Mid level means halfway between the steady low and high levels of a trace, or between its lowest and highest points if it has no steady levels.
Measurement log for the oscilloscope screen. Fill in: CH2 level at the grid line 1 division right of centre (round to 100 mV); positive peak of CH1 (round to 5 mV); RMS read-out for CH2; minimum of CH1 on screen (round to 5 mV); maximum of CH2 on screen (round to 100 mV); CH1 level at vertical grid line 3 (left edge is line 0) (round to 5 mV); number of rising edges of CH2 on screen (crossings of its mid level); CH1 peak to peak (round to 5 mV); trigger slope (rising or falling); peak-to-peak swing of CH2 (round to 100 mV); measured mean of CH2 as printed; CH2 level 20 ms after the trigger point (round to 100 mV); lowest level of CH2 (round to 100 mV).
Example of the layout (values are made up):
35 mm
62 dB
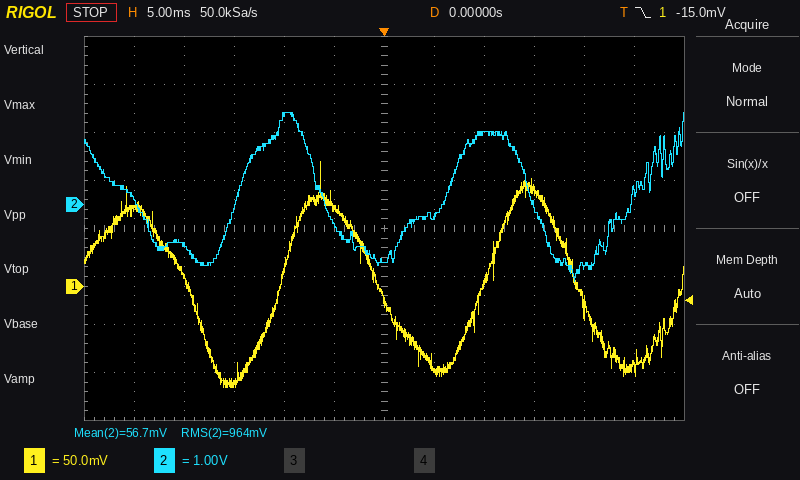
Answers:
-200 mV
130 mV
964 mV
-105 mV
1.9 V
-100 mV
3
235 mV
falling
3.5 V
56.7 mV
-1.3 V
-1.6 V
